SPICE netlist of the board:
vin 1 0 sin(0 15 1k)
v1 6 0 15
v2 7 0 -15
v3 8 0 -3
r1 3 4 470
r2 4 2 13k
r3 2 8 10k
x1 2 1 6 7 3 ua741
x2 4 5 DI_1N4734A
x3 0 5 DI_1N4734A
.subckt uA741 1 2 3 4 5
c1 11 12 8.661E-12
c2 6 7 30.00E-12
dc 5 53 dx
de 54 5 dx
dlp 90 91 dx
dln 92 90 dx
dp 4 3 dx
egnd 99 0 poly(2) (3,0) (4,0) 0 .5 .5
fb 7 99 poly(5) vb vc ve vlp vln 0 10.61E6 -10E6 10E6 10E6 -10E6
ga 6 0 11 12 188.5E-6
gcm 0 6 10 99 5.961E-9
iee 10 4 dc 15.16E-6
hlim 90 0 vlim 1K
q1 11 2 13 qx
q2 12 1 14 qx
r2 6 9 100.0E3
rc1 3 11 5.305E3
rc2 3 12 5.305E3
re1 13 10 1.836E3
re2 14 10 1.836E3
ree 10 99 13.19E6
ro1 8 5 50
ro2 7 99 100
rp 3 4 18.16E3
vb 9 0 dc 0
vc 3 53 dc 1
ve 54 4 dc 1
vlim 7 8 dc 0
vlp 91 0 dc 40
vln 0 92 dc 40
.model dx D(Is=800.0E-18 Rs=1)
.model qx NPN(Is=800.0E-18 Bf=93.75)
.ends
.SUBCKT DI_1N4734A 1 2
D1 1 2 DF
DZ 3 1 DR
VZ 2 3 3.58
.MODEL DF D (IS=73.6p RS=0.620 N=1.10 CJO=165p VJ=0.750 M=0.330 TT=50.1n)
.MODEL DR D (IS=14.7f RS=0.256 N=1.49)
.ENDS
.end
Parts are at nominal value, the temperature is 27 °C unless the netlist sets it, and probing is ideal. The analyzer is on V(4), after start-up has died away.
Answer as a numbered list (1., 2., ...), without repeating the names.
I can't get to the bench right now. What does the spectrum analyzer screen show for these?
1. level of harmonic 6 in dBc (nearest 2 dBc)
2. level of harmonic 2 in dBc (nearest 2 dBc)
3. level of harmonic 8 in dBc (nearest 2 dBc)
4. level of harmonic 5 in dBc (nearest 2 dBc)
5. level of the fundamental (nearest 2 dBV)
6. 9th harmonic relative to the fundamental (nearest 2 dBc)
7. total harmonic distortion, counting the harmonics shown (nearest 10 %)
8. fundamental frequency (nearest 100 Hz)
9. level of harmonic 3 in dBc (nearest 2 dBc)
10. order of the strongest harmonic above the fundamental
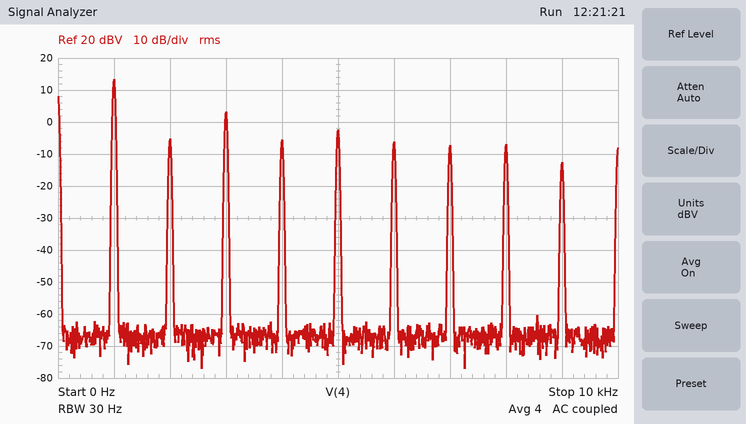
1. -20 dBc
2. -18 dBc
3. -20 dBc
4. -16 dBc
5. 14 dBV
6. -26 dBc
7. 40 %
8. 1.0 kHz
9. -10 dBc
10. 3
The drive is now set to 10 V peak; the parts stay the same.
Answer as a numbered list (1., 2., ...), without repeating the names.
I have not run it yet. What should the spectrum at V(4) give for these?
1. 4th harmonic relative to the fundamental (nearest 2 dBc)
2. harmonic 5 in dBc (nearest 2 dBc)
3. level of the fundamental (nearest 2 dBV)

1. -16 dBc
2. -18 dBc
3. 14 dBV
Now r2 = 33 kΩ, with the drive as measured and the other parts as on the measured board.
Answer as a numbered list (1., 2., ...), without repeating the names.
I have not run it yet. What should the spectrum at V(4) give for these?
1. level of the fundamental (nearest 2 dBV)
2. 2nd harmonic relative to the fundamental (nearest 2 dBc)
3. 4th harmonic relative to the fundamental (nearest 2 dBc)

1. 14 dBV
2. -16 dBc
3. -16 dBc
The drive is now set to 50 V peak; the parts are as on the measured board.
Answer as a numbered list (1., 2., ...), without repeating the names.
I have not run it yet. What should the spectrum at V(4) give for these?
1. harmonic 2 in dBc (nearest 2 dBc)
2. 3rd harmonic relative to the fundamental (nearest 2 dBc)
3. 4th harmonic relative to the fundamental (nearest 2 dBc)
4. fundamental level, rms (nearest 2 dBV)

1. 6 dBc
2. 0 dBc
3. 6 dBc
4. -6 dBV
